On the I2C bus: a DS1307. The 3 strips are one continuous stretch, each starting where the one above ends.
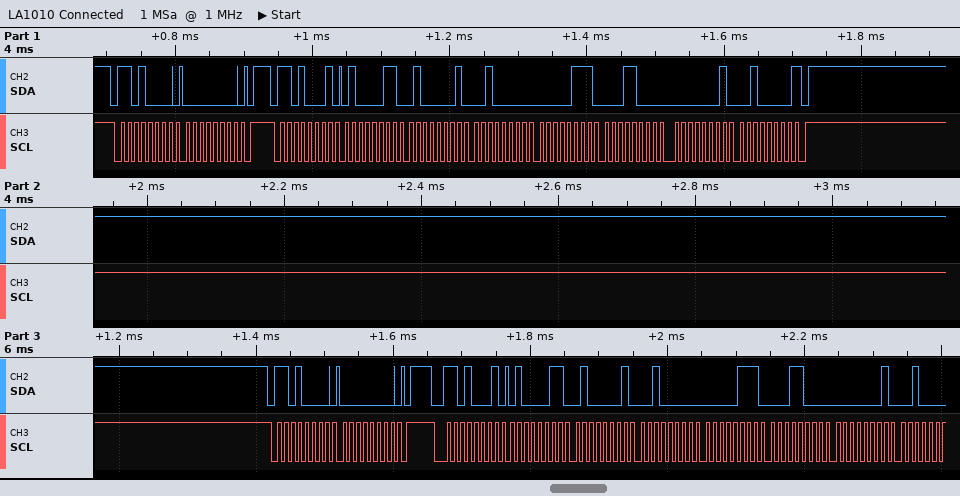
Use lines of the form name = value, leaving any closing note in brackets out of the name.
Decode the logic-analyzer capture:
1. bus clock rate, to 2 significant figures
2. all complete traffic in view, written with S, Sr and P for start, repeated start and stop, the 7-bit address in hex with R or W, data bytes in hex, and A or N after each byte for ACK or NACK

bus clock rate, to 2 significant figures = 100 kHz
all complete traffic in view, written with S, Sr and P for start, repeated start and stop, the 7-bit address in hex with R or W, data bytes in hex, and A or N after each byte for ACK or NACK = S 68W A 00 A P S 68R A 43 A 41 A 20 A 07 A 18 A 01 A 20 N P S 68W A 00 A P S 68R A 43 A 41 A 20 A 07 A 18 A 01 A
